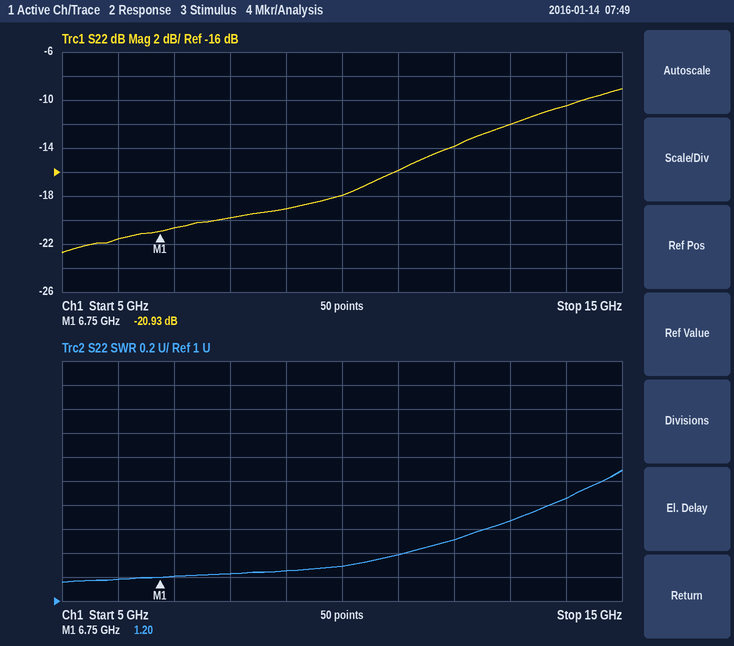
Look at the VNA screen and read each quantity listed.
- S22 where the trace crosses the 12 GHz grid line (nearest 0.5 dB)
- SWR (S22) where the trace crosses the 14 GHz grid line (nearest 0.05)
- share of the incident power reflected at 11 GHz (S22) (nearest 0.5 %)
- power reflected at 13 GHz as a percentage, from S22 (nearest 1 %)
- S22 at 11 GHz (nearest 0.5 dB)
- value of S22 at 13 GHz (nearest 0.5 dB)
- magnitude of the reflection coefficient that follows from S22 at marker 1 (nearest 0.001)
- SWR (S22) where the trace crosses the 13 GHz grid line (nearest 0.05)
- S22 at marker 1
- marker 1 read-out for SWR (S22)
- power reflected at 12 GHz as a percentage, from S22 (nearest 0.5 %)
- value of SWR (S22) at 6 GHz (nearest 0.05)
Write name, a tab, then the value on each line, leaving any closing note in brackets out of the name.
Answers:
S22 where the trace crosses the 12 GHz grid line	-14.0 dB
SWR (S22) where the trace crosses the 14 GHz grid line	1.85
share of the incident power reflected at 11 GHz (S22)	2.5 %
power reflected at 13 GHz as a percentage, from S22	6 %
S22 at 11 GHz	-16.0 dB
value of S22 at 13 GHz	-12.0 dB
magnitude of the reflection coefficient that follows from S22 at marker 1	0.090
SWR (S22) where the trace crosses the 13 GHz grid line	1.65
S22 at marker 1	-20.93 dB
marker 1 read-out for SWR	1.20
power reflected at 12 GHz as a percentage, from S22	4.0 %
value of SWR (S22) at 6 GHz	1.20
